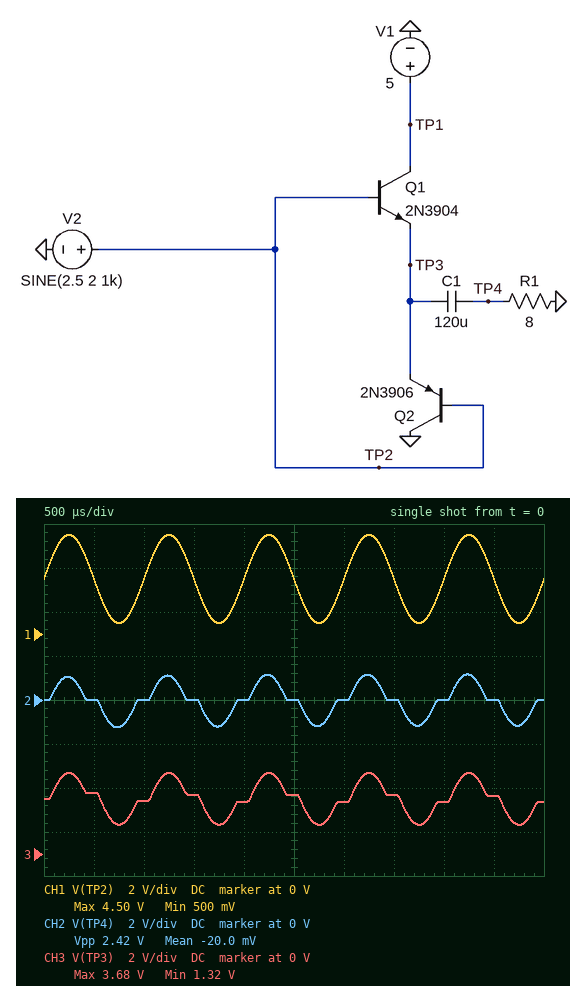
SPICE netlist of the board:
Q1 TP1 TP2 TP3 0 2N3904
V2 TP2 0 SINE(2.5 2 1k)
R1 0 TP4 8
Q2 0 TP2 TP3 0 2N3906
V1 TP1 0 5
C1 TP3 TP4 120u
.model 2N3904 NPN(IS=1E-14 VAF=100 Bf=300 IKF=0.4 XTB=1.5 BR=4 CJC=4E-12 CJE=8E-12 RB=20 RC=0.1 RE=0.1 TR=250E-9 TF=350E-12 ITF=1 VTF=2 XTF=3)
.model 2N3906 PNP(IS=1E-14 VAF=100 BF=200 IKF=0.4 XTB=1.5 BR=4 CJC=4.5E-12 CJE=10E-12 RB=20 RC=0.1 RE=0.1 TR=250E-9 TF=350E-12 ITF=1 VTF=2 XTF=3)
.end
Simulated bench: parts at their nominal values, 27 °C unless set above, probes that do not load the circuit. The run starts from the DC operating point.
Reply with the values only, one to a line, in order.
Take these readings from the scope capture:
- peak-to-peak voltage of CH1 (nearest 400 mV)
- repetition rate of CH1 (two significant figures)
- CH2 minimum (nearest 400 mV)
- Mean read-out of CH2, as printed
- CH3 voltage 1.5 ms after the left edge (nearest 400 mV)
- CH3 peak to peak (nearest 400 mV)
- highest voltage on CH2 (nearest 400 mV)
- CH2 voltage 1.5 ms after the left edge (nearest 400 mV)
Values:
4.0 V
1.0 kHz
-1.2 V
-20.0 mV
2.8 V
2.4 V
1.2 V
0 V
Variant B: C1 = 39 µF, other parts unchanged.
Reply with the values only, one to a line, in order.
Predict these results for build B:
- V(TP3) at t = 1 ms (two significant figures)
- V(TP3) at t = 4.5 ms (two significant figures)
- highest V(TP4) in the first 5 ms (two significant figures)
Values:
2.1 V
2.9 V
1.1 V
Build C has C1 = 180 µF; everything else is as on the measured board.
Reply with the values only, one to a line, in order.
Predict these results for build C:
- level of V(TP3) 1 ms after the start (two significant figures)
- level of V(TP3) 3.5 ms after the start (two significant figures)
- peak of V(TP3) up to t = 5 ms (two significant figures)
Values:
2.5 V
2.6 V
3.7 V
